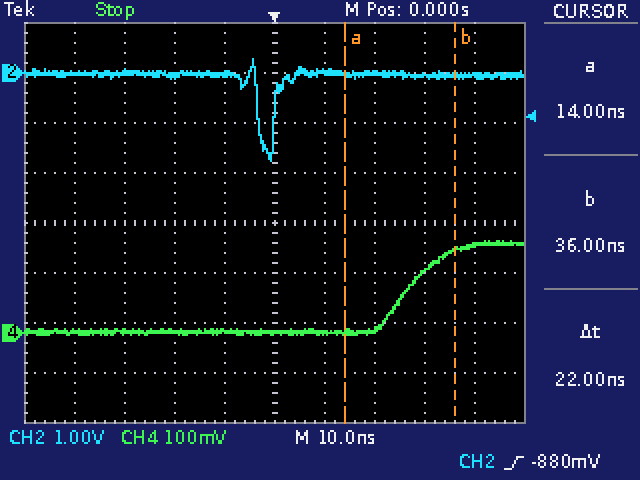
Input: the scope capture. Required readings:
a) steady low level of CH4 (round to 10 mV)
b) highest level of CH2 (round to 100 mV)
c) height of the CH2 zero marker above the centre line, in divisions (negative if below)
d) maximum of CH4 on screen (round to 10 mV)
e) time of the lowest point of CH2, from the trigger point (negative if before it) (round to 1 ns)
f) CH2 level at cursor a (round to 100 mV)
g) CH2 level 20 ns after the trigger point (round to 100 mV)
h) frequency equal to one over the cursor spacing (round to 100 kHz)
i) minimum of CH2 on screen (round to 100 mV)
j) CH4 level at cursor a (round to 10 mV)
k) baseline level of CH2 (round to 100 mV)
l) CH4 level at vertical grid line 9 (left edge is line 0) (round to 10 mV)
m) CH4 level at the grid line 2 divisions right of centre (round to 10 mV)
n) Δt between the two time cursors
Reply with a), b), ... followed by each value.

a) 0 mV
b) 300 mV
c) +3.0 div
d) 180 mV
e) -1 ns
f) 0.0 V
g) 0.0 V
h) 45.5 MHz
i) -1.8 V
j) 0 mV
k) 0.0 V
l) 180 mV
m) 10 mV
n) 22 ns
